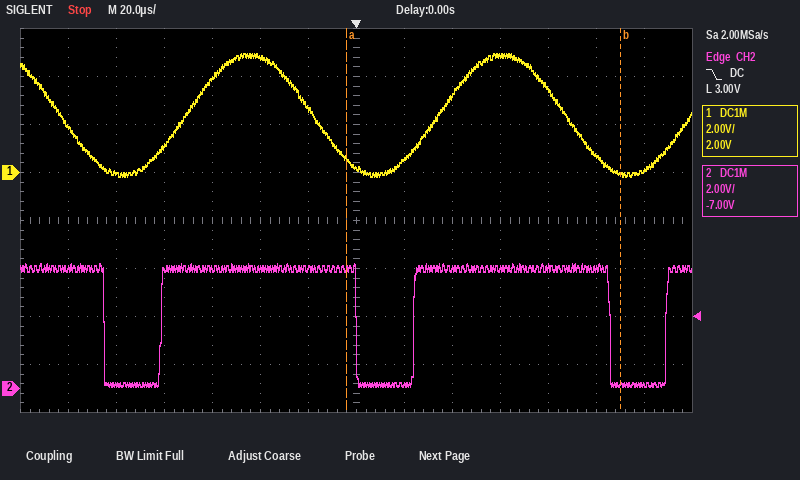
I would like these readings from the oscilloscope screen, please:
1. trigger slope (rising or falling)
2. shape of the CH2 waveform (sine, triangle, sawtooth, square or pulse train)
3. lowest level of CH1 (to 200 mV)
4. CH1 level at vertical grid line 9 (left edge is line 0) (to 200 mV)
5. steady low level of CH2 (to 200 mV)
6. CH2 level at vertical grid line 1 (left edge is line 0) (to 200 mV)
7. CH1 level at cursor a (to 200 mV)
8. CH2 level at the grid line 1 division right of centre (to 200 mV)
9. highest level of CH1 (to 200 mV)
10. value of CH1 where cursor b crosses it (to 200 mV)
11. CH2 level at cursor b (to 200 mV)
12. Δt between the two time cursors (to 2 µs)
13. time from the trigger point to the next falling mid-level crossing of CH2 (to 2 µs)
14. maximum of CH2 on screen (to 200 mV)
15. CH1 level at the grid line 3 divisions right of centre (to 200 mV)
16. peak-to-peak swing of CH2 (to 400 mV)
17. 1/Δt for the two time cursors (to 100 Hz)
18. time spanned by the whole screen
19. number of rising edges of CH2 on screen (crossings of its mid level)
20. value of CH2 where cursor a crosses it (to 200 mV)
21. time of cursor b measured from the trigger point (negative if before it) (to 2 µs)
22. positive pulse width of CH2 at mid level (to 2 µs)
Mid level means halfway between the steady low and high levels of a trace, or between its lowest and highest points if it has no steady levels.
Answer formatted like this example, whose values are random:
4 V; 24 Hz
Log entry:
falling; pulse train; -200 mV; 3.2 V; 200 mV; 5.0 V; 600 mV; 200 mV; 5.0 V; 0.0 V; 200 mV; 114 µs; 106 µs; 5.2 V; 4.8 V; 5.2 V; 8.8 kHz; 280 µs; 3; 5.0 V; +110 µs; 82 µs
